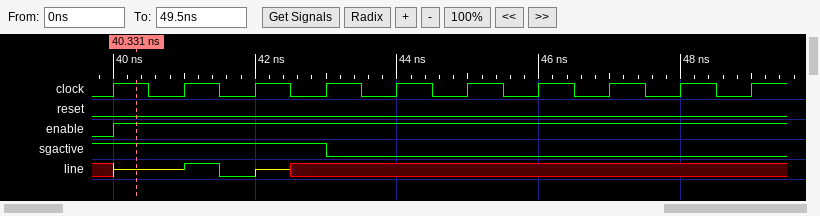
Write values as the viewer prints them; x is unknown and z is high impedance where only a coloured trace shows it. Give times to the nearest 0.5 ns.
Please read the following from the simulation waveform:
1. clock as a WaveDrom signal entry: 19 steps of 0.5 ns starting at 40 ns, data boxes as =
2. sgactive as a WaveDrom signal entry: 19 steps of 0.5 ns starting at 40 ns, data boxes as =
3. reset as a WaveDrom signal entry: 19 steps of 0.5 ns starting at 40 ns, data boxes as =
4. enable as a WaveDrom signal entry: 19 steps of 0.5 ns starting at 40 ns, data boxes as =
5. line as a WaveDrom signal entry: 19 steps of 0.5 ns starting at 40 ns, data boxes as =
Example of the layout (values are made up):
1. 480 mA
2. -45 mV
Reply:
1. {name: 'clock', wave: '1010101010101010101'}
2. {name: 'sgactive', wave: '1.....0............'}
3. {name: 'reset', wave: '0..................'}
4. {name: 'enable', wave: '1..................'}
5. {name: 'line', wave: 'z.10zx.............'}
